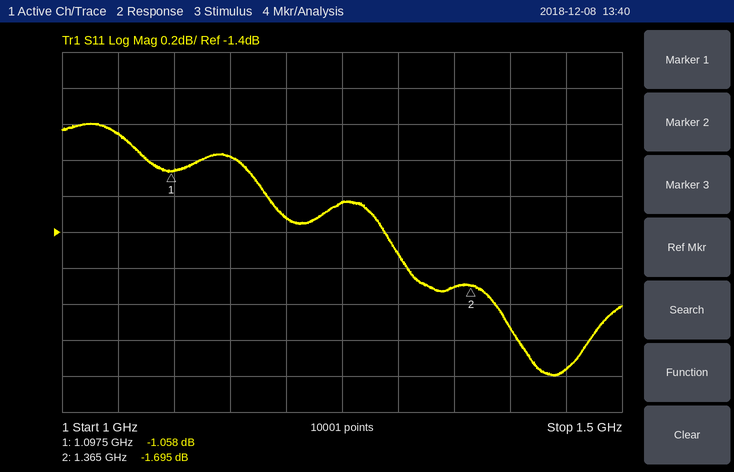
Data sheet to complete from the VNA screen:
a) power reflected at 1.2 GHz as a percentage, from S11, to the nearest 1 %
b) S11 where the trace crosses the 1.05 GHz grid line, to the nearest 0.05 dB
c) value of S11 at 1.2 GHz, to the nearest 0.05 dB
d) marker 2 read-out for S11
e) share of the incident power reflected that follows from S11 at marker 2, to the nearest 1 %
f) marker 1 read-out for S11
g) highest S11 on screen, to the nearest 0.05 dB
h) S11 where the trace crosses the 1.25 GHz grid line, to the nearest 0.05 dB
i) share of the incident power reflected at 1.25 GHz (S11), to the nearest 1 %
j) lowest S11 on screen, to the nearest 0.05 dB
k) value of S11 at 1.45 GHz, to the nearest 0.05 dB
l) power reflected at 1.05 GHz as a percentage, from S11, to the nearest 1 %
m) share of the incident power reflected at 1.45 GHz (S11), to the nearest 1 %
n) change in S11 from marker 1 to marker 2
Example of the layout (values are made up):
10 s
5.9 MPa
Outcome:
74 %
-0.85 dB
-1.30 dB
-1.695 dB
68 %
-1.058 dB
-0.80 dB
-1.25 dB
75 %
-2.20 dB
-2.15 dB
82 %
61 %
-0.637 dB
